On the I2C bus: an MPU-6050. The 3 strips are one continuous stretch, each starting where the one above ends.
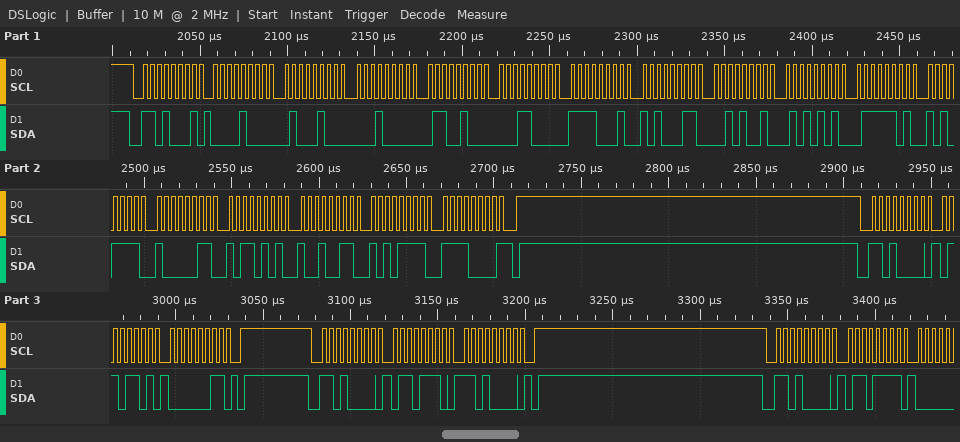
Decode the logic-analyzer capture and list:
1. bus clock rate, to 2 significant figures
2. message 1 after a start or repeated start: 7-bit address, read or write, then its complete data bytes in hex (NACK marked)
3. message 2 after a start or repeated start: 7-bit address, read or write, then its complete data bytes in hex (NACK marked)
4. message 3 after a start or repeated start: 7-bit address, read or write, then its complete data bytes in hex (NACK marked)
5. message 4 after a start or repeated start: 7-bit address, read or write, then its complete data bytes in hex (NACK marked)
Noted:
250 kHz
0x68 read: 08 44 10 64 18 F1 A3 29 55 7D AF 83 B5 93 AF F0 NACK
0x68 write: 6D 03
0x68 write: 6E D0
0x68 write: 6F
